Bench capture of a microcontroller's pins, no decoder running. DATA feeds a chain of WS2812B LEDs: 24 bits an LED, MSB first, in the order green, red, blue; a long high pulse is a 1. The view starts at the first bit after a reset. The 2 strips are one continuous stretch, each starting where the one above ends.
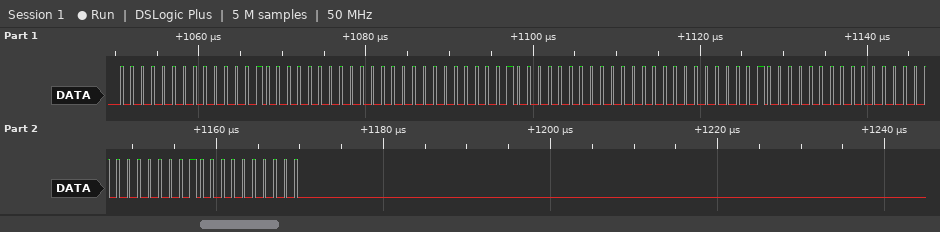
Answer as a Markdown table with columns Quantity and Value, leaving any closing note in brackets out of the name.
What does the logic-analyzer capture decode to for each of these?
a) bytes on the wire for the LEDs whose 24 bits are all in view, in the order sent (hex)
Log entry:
| Quantity | Value |
|---|---|
| bytes on the wire for the LEDs whose 24 bits are all in view, in the order sent | 00 04 00 00 04 00 00 04 00 00 04 00 |
